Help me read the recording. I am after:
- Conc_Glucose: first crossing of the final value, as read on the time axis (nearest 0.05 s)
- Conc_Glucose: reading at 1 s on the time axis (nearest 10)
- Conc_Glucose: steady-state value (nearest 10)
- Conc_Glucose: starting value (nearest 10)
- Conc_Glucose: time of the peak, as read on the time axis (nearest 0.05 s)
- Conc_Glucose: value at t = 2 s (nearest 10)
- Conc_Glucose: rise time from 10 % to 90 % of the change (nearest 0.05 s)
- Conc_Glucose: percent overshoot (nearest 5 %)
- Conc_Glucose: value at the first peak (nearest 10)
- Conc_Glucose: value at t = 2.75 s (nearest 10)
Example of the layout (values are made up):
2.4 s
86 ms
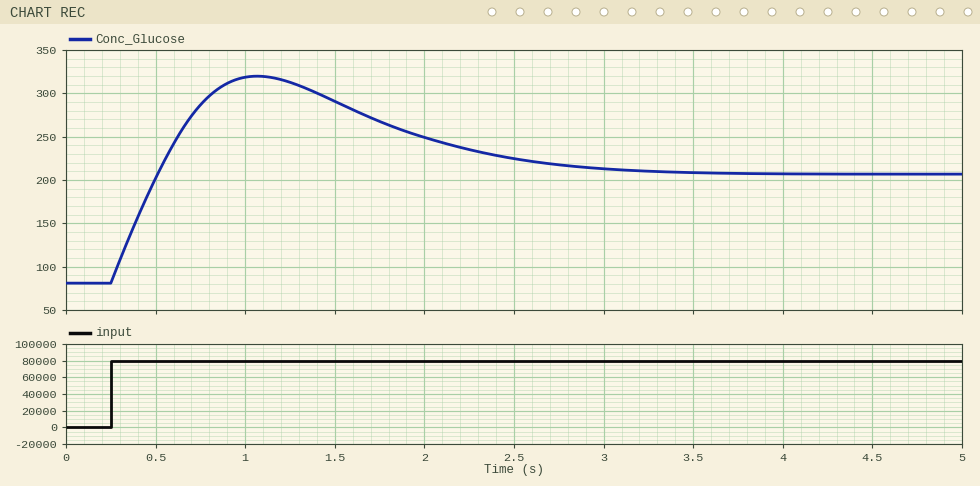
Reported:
0.50 s
320
210
80
1.05 s
250
0.20 s
90 %
320
220
